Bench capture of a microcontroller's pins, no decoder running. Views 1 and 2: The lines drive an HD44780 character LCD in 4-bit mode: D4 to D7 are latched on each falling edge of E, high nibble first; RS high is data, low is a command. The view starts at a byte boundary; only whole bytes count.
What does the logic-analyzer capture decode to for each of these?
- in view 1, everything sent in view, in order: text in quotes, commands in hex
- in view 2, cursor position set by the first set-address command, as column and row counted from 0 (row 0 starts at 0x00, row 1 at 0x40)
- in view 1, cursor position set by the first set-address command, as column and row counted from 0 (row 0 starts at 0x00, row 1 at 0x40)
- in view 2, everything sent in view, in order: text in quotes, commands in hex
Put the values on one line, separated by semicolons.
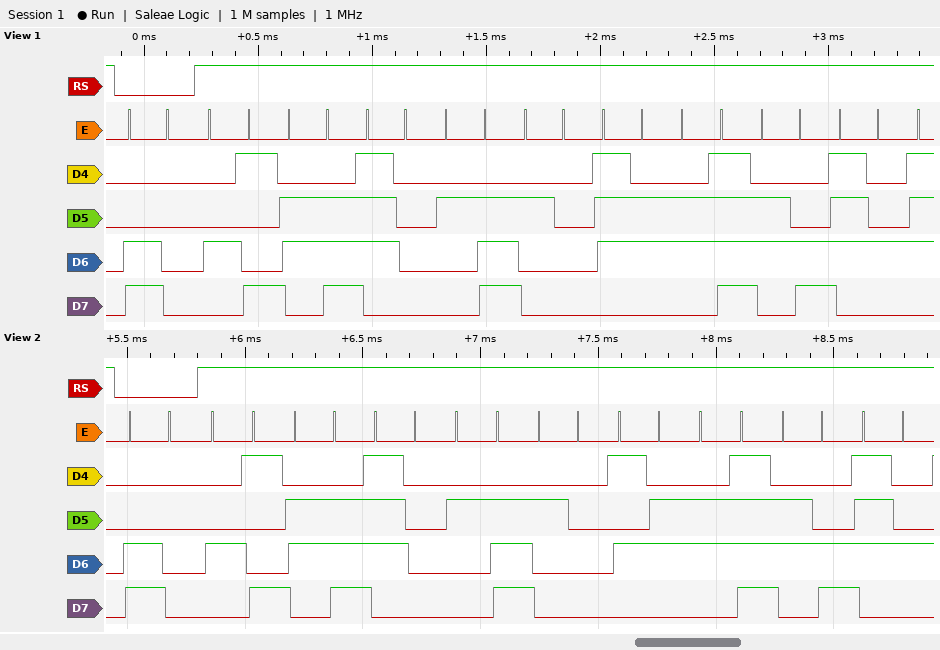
0xC0 "Inp. volt"; column 0, row 1; column 0, row 1; 0xC0 "Inp. Volt"
